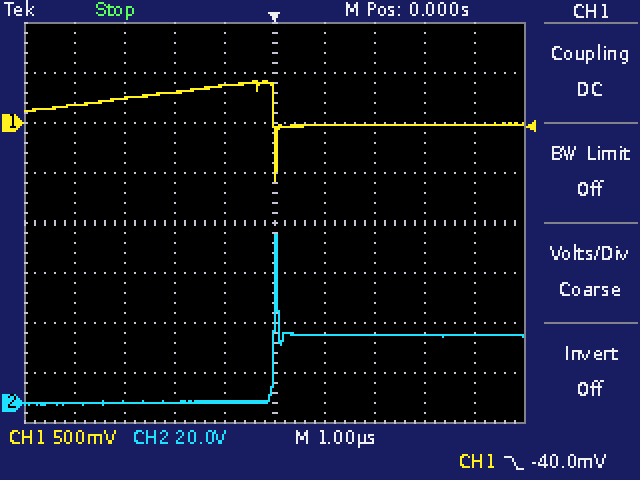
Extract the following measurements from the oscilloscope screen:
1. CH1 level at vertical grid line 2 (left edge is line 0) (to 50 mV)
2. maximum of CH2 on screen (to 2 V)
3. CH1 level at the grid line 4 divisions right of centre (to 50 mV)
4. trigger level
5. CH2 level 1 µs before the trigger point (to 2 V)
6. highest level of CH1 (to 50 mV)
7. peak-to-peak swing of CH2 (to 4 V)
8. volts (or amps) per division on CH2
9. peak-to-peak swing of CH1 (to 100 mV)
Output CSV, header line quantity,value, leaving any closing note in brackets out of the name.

quantity,value
CH1 level at vertical grid line 2 (left edge is line 0),250 mV
maximum of CH2 on screen,68 V
CH1 level at the grid line 4 divisions right of centre,0 mV
trigger level,-40.0 mV
CH2 level 1 µs before the trigger point,0 V
highest level of CH1,400 mV
peak-to-peak swing of CH2,68 V
volts (or amps) per division on CH2,20 V
peak-to-peak swing of CH1,1.00 V
